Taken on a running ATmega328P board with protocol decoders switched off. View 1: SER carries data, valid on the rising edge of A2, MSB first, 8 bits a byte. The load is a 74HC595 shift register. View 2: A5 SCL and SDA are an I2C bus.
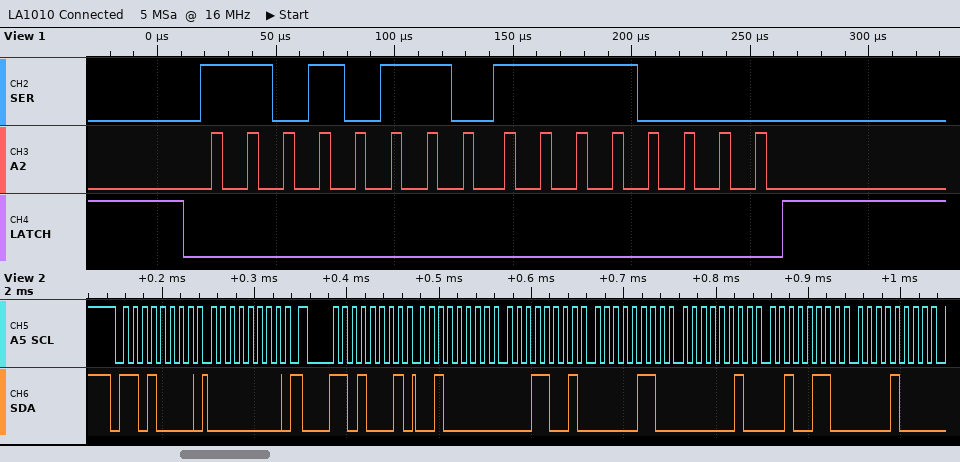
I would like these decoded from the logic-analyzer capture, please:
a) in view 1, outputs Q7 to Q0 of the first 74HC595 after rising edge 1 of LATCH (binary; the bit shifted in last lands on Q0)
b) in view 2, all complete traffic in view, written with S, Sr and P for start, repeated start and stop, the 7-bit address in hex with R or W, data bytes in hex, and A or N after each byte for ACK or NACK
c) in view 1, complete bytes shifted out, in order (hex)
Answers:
11110000
S 68W A 00 A Sr 68R A 20 A 19 A 06 A 02 A 26 A 08 A
D6 F0
